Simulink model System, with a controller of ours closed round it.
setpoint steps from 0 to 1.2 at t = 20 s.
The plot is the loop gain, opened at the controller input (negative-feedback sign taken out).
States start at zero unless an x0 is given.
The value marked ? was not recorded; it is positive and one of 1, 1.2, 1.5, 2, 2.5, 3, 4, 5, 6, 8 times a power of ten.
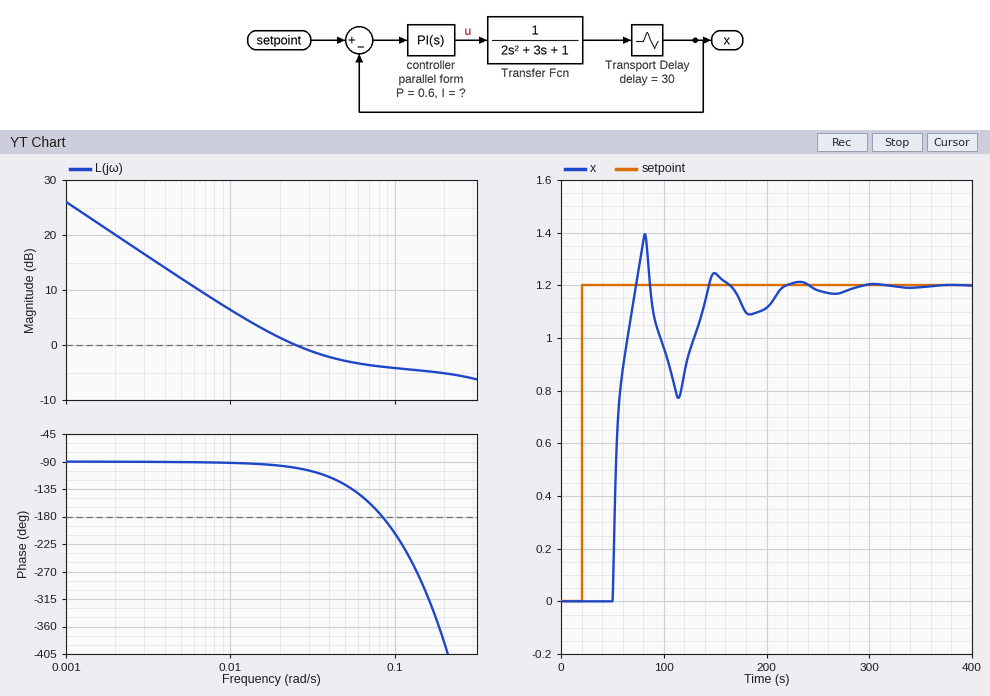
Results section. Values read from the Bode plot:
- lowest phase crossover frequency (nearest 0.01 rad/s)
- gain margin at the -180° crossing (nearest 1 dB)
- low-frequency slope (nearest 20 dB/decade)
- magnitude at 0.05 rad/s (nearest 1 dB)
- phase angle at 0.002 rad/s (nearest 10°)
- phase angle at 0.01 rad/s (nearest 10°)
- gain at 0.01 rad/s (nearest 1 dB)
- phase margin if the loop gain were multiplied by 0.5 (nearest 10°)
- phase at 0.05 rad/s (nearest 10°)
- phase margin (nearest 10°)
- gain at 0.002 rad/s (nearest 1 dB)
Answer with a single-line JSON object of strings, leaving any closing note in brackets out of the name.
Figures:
{"lowest phase crossover frequency": "0.08 rad/s", "gain margin at the -180° crossing": "4 dB", "low-frequency slope": "-20 dB/decade", "magnitude at 0.05 rad/s": "-3 dB", "phase angle at 0.002 rad/s": "-90°", "phase angle at 0.01 rad/s": "-90°", "gain at 0.01 rad/s": "6 dB", "phase margin if the loop gain were multiplied by 0.5": "90°", "phase at 0.05 rad/s": "-130°", "phase margin": "80°", "gain at 0.002 rad/s": "20 dB"}
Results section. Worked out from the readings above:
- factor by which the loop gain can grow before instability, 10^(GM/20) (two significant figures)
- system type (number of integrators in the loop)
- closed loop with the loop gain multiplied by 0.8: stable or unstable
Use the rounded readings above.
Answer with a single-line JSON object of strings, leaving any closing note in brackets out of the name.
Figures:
{"factor by which the loop gain can grow before instability, 10^(GM/20)": "1.6", "system type": "1", "closed loop with the loop gain multiplied by 0.8: stable or unstable": "stable"}
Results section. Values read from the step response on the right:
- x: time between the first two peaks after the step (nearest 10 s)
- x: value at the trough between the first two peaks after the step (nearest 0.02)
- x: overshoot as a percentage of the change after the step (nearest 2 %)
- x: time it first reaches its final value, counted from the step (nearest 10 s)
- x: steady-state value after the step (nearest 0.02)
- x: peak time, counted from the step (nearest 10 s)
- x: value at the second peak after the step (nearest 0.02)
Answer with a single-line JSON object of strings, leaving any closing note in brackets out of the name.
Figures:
{"x: time between the first two peaks after the step": "70 s", "x: value at the trough between the first two peaks after the step": "0.78", "x: overshoot as a percentage of the change after the step": "16 %", "x: time it first reaches its final value, counted from the step": "50 s", "x: steady-state value after the step": "1.20", "x: peak time, counted from the step": "60 s", "x: value at the second peak after the step": "1.24"}
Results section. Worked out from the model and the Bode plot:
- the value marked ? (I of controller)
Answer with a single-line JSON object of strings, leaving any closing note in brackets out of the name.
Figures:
{"the value marked ?": "0.02"}
